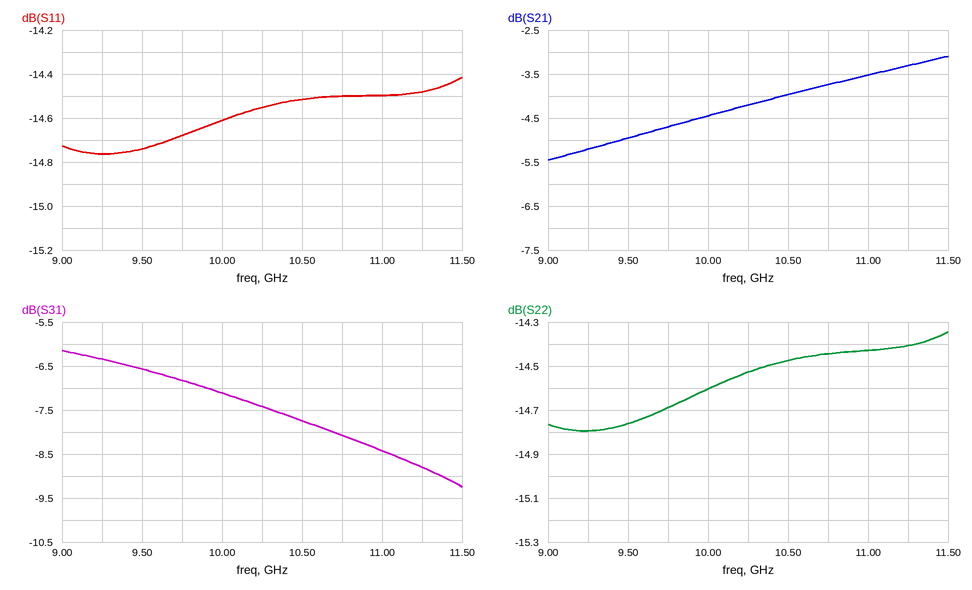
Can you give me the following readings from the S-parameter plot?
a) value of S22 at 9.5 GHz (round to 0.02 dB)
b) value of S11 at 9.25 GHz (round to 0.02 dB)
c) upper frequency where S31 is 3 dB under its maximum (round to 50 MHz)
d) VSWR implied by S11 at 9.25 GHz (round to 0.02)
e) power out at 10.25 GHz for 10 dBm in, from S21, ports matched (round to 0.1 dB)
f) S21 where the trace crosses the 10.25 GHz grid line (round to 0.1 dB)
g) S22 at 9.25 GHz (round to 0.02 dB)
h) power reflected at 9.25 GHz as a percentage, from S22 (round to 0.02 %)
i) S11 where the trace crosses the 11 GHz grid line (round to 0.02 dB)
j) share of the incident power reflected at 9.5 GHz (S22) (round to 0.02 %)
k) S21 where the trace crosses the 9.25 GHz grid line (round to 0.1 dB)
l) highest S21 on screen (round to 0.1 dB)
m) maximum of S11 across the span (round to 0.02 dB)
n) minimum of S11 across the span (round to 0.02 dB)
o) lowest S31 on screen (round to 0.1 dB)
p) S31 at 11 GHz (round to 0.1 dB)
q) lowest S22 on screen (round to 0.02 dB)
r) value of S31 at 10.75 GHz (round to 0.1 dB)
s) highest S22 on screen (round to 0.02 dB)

-14.76 dB
-14.76 dB
11.45 GHz
1.44
5.8 dBm
-4.2 dB
-14.80 dB
3.32 %
-14.50 dB
3.34 %
-5.2 dB
-3.1 dB
-14.42 dB
-14.76 dB
-9.2 dB
-8.4 dB
-14.80 dB
-8.1 dB
-14.34 dB
